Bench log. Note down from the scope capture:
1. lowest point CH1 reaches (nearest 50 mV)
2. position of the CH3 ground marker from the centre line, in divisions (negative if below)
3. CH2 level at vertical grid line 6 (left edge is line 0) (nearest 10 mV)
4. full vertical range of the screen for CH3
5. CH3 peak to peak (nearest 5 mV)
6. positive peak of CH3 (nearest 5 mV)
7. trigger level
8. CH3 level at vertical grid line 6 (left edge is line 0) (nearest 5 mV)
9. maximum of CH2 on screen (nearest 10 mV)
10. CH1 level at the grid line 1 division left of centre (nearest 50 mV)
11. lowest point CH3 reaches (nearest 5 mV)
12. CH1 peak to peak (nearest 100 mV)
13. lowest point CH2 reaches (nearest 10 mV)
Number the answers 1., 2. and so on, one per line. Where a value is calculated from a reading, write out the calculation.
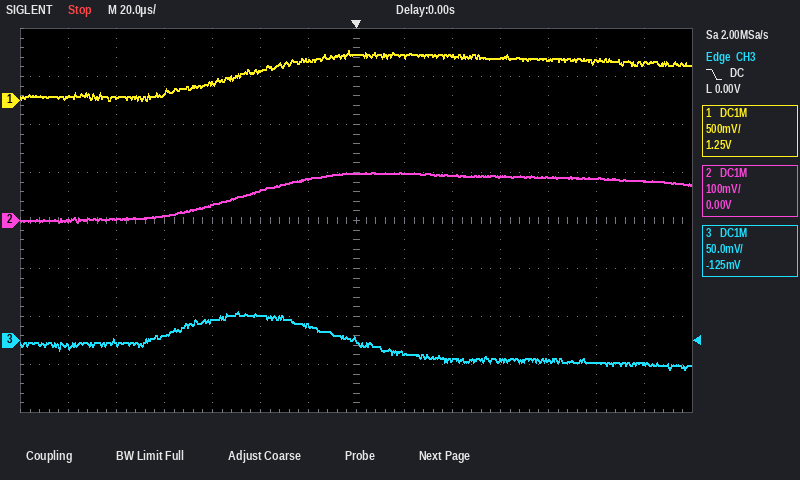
1. 0 mV
2. -2.5 div
3. 90 mV
4. 400 mV
5. 30 mV − (-30 mV) = 60 mV
6. 30 mV
7. 0.00 V
8. 15 mV
9. 100 mV
10. 400 mV
11. -30 mV
12. 500 mV
13. 0 mV
